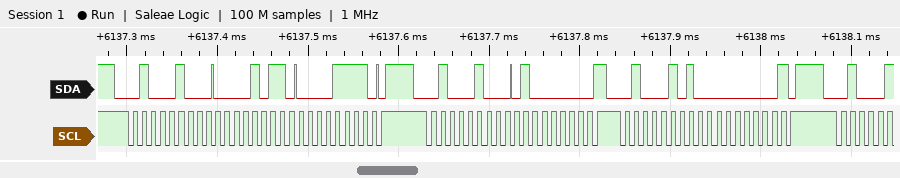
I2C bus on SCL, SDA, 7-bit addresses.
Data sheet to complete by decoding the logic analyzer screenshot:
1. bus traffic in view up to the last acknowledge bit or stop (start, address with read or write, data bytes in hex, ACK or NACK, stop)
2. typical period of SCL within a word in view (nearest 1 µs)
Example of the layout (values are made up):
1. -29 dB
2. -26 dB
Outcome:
1. start, address 22 write ACK, 0B ACK, 0F ACK, stop, start, address 22 write ACK, 40 ACK, repeated start, address 22 read ACK, 00 NACK, stop
2. 10 µs
